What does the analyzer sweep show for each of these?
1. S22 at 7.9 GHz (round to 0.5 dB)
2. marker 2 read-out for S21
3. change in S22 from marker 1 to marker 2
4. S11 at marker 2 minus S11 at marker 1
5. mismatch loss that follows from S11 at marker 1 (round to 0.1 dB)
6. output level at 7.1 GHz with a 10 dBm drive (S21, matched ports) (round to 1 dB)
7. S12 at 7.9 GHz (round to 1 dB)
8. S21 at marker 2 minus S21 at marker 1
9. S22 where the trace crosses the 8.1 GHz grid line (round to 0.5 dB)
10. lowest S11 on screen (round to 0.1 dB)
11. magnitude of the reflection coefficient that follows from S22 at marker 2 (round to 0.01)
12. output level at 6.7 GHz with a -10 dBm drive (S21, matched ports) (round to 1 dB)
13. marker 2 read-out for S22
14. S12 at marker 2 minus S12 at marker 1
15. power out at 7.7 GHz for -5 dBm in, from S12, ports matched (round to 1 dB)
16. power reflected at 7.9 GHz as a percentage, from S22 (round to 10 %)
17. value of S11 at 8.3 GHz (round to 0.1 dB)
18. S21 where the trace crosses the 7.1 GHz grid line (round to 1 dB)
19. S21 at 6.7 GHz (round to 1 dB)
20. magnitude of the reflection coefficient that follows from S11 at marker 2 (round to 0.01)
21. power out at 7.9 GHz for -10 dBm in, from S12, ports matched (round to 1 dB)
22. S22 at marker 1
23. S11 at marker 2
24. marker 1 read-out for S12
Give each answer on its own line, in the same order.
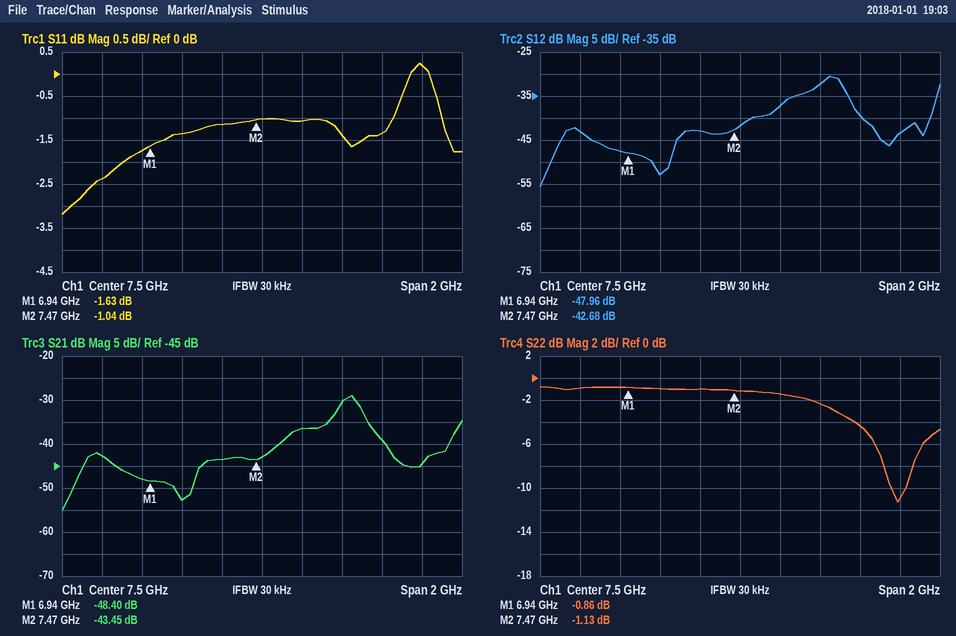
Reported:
-2.5 dB
-43.45 dB
-0.27 dB
0.59 dB
5.0 dB
-43 dBm
-32 dB
4.95 dB
-4.5 dB
-3.2 dB
0.88
-53 dBm
-1.13 dB
5.28 dB
-42 dBm
60 %
0.2 dB
-53 dB
-43 dB
0.89
-42 dBm
-0.86 dB
-1.04 dB
-47.96 dB
